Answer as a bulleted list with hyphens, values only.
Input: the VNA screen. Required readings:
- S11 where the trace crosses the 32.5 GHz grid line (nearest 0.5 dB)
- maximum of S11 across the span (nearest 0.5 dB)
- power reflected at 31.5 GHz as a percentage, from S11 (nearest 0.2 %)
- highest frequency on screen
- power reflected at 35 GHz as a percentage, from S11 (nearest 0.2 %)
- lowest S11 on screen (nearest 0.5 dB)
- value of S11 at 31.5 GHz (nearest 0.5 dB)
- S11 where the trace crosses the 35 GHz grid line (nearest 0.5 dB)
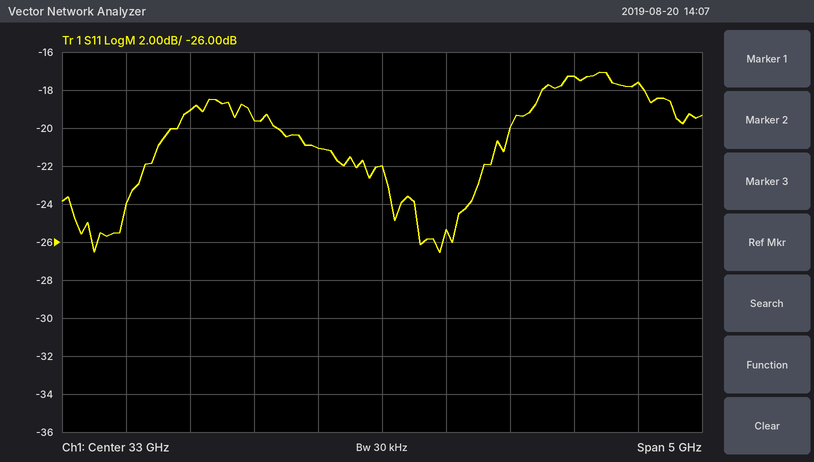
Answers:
- -21.0 dB
- -17.0 dB
- 1.2 %
- 35.5 GHz
- 1.8 %
- -26.5 dB
- -19.0 dB
- -17.5 dB
